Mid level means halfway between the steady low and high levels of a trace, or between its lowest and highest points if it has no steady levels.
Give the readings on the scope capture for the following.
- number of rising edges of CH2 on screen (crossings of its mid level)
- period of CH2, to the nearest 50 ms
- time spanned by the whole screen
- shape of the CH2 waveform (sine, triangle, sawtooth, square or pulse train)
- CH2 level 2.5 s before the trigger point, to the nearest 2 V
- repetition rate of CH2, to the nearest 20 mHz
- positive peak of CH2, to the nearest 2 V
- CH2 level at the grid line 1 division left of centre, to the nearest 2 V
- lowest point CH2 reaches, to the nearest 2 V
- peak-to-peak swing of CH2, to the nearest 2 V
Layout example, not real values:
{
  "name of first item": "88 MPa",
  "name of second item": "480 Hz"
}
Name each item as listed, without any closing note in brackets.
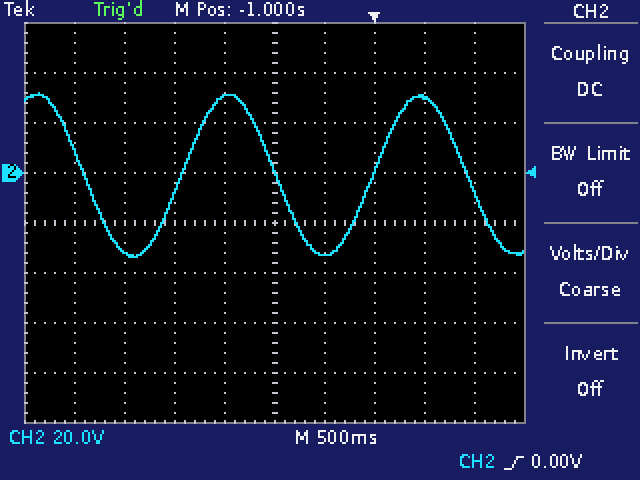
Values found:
{
  "number of rising edges of CH2 on screen": "2",
  "period of CH2, to the nearest 50 ms": "1.90 s",
  "time spanned by the whole screen": "5 s",
  "shape of the CH2 waveform": "sine",
  "CH2 level 2.5 s before the trigger point, to the nearest 2 V": "-32 V",
  "repetition rate of CH2, to the nearest 20 mHz": "520 mHz",
  "positive peak of CH2, to the nearest 2 V": "32 V",
  "CH2 level at the grid line 1 division left of centre, to the nearest 2 V": "30 V",
  "lowest point CH2 reaches, to the nearest 2 V": "-34 V",
  "peak-to-peak swing of CH2, to the nearest 2 V": "66 V"
}
